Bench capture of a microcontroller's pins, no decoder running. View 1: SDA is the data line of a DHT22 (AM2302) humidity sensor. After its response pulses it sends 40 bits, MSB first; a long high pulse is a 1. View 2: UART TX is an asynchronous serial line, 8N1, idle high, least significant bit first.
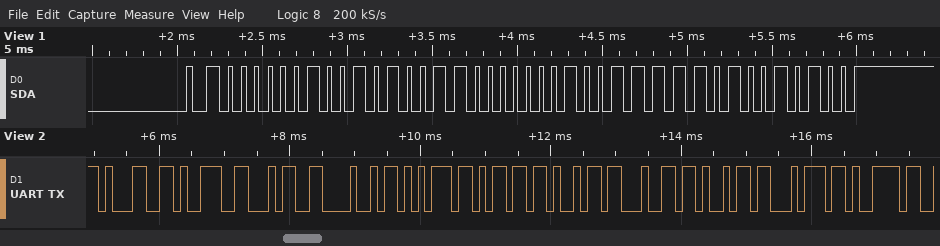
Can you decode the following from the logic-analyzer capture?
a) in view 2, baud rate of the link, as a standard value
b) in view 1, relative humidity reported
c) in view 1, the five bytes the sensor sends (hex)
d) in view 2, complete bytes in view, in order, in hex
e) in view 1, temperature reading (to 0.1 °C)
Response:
9600 baud
59.5 %
02 53 01 3E 94
31 39 34 48 75 6D 69 64 69 74 79
31.8 °C
